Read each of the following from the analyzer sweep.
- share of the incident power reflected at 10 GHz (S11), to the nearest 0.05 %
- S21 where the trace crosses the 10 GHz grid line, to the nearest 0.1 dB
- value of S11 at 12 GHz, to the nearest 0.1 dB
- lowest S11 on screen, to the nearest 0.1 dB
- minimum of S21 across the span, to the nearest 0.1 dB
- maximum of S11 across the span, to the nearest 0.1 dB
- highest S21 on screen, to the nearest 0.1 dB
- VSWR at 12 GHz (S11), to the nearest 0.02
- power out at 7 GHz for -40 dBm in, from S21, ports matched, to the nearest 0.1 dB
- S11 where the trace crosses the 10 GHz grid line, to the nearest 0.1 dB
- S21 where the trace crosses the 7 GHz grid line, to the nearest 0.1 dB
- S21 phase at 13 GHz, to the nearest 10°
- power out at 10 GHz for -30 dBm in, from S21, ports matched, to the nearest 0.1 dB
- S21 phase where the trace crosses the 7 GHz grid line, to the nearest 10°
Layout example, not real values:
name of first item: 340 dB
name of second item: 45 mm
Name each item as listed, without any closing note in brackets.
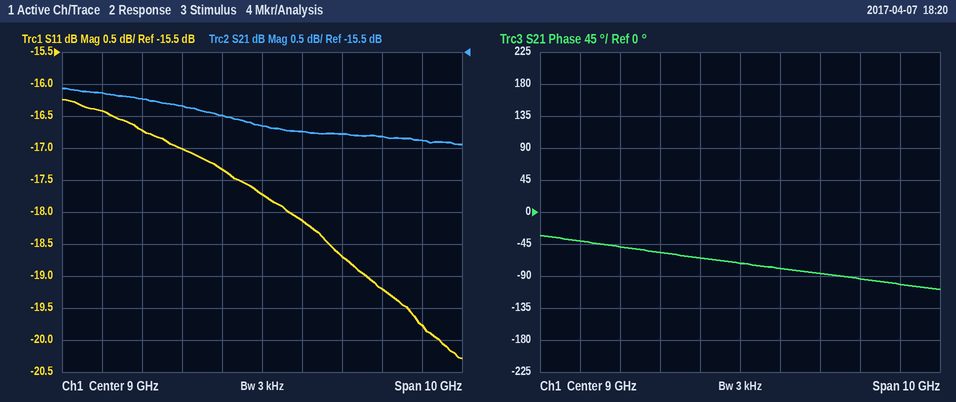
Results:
share of the incident power reflected at 10 GHz (S11), to the nearest 0.05 %: 1.55 %
S21 where the trace crosses the 10 GHz grid line, to the nearest 0.1 dB: -16.7 dB
value of S11 at 12 GHz, to the nearest 0.1 dB: -19.2 dB
lowest S11 on screen, to the nearest 0.1 dB: -20.3 dB
minimum of S21 across the span, to the nearest 0.1 dB: -16.9 dB
maximum of S11 across the span, to the nearest 0.1 dB: -16.2 dB
highest S21 on screen, to the nearest 0.1 dB: -16.1 dB
VSWR at 12 GHz (S11), to the nearest 0.02: 1.24
power out at 7 GHz for -40 dBm in, from S21, ports matched, to the nearest 0.1 dB: -56.3 dBm
S11 where the trace crosses the 10 GHz grid line, to the nearest 0.1 dB: -18.1 dB
S21 where the trace crosses the 7 GHz grid line, to the nearest 0.1 dB: -16.3 dB
S21 phase at 13 GHz, to the nearest 10°: -100°
power out at 10 GHz for -30 dBm in, from S21, ports matched, to the nearest 0.1 dB: -46.7 dBm
S21 phase where the trace crosses the 7 GHz grid line, to the nearest 10°: -60°
